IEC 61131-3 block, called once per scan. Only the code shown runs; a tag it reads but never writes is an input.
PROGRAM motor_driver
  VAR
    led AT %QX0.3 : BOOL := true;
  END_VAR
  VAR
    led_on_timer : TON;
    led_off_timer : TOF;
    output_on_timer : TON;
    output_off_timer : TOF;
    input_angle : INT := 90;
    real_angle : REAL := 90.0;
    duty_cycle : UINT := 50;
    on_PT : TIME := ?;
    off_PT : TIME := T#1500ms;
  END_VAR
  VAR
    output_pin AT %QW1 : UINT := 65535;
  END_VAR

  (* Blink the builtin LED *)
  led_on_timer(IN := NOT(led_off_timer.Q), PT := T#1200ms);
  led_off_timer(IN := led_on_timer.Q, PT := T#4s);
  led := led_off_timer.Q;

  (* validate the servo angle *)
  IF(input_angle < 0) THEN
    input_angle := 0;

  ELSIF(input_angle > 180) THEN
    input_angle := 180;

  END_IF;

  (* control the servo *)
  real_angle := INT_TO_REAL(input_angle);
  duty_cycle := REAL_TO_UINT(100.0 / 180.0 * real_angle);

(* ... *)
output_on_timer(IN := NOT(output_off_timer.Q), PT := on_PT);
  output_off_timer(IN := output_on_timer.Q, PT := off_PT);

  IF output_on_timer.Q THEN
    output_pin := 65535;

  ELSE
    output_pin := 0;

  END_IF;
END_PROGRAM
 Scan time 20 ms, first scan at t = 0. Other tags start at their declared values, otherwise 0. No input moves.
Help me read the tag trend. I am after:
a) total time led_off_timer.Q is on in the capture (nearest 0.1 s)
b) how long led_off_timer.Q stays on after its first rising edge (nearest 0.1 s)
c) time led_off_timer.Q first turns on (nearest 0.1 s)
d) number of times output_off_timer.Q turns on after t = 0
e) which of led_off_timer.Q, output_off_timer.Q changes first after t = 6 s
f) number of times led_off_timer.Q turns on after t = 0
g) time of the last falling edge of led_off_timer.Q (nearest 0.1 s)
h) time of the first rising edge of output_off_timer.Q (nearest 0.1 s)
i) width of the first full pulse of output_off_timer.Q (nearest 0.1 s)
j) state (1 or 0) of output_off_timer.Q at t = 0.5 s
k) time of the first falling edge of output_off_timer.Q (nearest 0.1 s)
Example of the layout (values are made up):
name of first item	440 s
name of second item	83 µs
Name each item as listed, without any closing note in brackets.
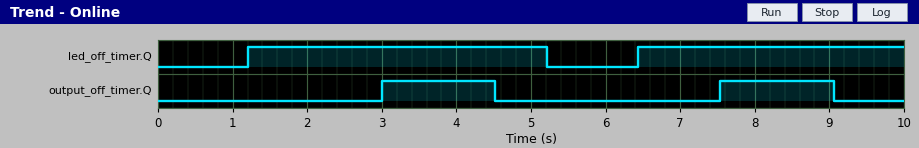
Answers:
total time led_off_timer.Q is on in the capture	7.6 s
how long led_off_timer.Q stays on after its first rising edge	4.0 s
time led_off_timer.Q first turns on	1.2 s
number of times output_off_timer.Q turns on after t = 0	2
which of led_off_timer.Q, output_off_timer.Q changes first after t = 6 s	led_off_timer.Q
number of times led_off_timer.Q turns on after t = 0	2
time of the last falling edge of led_off_timer.Q	5.2 s
time of the first rising edge of output_off_timer.Q	3.0 s
width of the first full pulse of output_off_timer.Q	1.5 s
state (1 or 0) of output_off_timer.Q at t = 0.5 s	0
time of the first falling edge of output_off_timer.Q	4.5 s
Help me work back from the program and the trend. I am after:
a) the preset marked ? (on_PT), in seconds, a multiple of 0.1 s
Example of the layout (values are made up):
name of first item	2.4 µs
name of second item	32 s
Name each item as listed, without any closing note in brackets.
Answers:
the preset marked ? (on_PT), in seconds, a multiple of 0.1 s	3.0 s
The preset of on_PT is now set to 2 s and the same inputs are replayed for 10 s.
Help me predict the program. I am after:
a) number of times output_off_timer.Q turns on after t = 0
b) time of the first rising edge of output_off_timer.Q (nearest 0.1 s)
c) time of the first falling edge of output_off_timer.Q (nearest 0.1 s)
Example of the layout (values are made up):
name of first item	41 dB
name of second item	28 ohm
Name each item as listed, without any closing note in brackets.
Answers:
number of times output_off_timer.Q turns on after t = 0	3
time of the first rising edge of output_off_timer.Q	2.0 s
time of the first falling edge of output_off_timer.Q	3.5 s
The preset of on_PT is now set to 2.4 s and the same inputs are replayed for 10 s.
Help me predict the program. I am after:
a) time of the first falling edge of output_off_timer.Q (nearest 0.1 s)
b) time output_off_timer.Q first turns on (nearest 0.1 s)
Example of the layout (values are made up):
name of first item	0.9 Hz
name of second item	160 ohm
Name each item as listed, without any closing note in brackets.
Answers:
time of the first falling edge of output_off_timer.Q	3.9 s
time output_off_timer.Q first turns on	2.4 s
